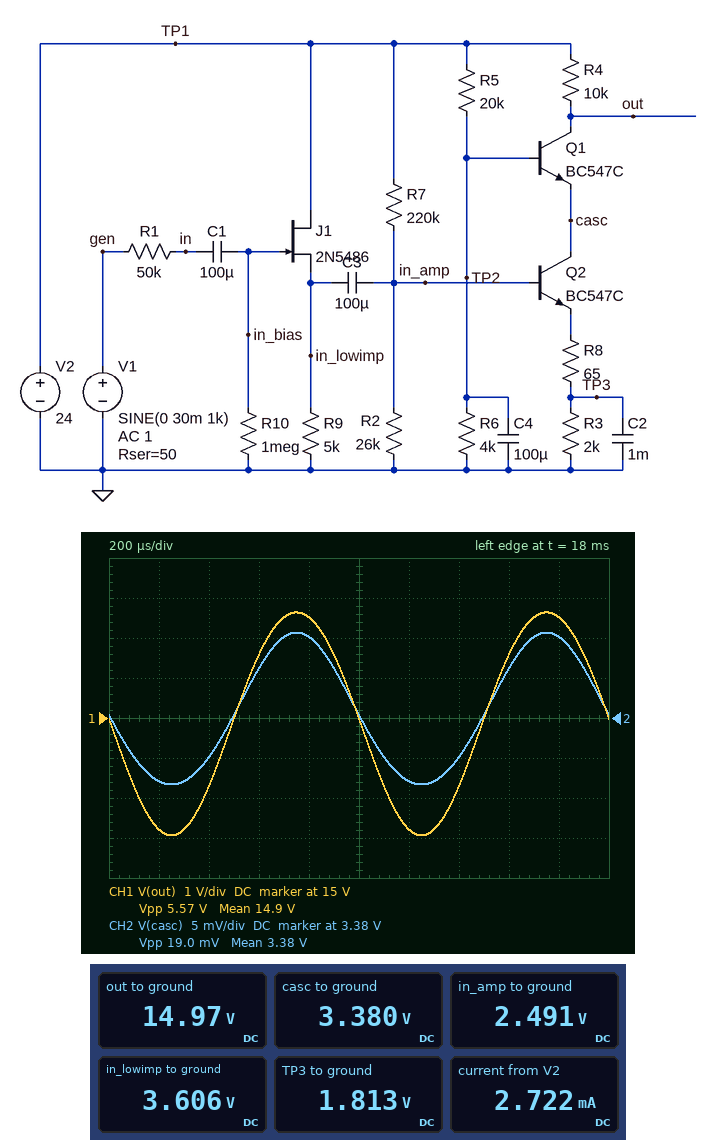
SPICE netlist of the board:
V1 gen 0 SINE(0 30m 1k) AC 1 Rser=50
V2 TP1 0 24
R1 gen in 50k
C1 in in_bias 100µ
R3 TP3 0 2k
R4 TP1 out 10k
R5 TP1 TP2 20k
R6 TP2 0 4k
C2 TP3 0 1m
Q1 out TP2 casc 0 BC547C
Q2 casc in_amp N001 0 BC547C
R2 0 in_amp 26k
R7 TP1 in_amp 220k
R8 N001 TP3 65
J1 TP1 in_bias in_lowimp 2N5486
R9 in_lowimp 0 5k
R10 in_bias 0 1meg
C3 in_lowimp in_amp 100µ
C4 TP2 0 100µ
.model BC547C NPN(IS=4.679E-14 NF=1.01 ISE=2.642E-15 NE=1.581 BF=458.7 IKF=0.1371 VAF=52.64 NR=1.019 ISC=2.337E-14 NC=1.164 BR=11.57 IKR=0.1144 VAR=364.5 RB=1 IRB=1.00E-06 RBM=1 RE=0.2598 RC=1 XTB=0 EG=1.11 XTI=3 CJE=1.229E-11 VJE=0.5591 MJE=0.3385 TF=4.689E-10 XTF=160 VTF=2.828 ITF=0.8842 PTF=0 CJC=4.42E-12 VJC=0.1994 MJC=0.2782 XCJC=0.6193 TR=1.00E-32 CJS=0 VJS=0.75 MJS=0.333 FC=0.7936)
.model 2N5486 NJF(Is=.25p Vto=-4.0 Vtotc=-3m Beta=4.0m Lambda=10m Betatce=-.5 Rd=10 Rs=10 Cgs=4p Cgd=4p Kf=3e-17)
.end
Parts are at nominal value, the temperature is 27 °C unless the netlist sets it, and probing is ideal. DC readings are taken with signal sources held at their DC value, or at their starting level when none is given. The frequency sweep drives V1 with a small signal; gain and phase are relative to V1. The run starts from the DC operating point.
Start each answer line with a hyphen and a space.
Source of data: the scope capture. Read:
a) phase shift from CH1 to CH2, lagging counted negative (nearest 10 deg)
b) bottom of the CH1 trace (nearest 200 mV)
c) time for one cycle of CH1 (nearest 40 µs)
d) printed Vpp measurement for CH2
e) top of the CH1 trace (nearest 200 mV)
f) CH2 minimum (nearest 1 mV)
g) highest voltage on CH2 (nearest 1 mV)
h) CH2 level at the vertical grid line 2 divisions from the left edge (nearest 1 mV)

- 0 deg
- 12.0 V
- 1.00 ms
- 19.0 mV
- 17.6 V
- 3.372 V
- 3.391 V
- 3.375 V
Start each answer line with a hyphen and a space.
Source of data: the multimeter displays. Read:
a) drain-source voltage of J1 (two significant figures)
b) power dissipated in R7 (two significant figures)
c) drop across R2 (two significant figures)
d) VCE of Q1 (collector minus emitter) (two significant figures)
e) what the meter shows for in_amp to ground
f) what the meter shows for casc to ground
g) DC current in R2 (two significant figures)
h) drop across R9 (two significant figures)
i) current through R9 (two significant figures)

- 20 V
- 2.1 mW
- 2.5 V
- 12 V
- 2.491 V
- 3.380 V
- 96 µA
- 3.6 V
- 720 µA
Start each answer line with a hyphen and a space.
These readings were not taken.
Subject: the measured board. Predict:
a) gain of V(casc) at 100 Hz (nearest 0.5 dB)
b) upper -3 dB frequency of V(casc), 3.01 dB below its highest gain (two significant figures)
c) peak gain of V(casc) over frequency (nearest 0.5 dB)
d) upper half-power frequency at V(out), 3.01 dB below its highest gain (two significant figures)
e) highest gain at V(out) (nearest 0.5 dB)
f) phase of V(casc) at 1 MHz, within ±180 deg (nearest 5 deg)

- -10.0 dB
- 4.0 MHz
- -10.0 dB
- 3.7 MHz
- 39.5 dB
- 160 deg
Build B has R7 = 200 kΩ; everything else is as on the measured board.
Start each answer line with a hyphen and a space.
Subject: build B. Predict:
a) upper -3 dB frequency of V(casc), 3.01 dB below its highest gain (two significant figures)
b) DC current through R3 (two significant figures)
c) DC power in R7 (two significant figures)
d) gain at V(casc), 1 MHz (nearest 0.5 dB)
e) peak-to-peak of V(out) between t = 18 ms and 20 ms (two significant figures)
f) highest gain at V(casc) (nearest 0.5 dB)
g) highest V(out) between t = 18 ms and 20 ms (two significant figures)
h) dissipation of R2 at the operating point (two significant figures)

- 4.0 MHz
- 1.0 mA
- 2.3 mW
- -11.0 dB
- 5.8 V
- -10.5 dB
- 17 V
- 280 µW
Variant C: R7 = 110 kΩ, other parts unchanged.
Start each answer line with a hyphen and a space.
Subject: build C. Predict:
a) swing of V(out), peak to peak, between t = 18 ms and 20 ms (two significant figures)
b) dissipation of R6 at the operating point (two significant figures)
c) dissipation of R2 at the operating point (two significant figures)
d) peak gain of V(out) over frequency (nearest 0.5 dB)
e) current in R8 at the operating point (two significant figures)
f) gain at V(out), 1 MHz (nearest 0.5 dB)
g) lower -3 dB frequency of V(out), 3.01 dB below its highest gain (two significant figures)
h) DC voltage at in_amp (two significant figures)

- 3.8 V
- 4.0 mW
- 600 µW
- 36.0 dB
- 1.6 mA
- 35.5 dB
- 2.8 Hz
- 3.9 V
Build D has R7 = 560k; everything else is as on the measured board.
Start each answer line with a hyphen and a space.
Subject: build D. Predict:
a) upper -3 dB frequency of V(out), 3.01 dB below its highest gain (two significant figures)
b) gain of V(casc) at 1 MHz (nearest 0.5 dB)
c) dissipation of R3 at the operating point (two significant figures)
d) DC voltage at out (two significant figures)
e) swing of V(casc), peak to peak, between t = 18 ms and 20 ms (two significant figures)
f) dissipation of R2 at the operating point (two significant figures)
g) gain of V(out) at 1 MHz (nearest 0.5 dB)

- 3.8 MHz
- -5.0 dB
- 100 µW
- 22 V
- 35 mV
- 43 µW
- 33.5 dB
